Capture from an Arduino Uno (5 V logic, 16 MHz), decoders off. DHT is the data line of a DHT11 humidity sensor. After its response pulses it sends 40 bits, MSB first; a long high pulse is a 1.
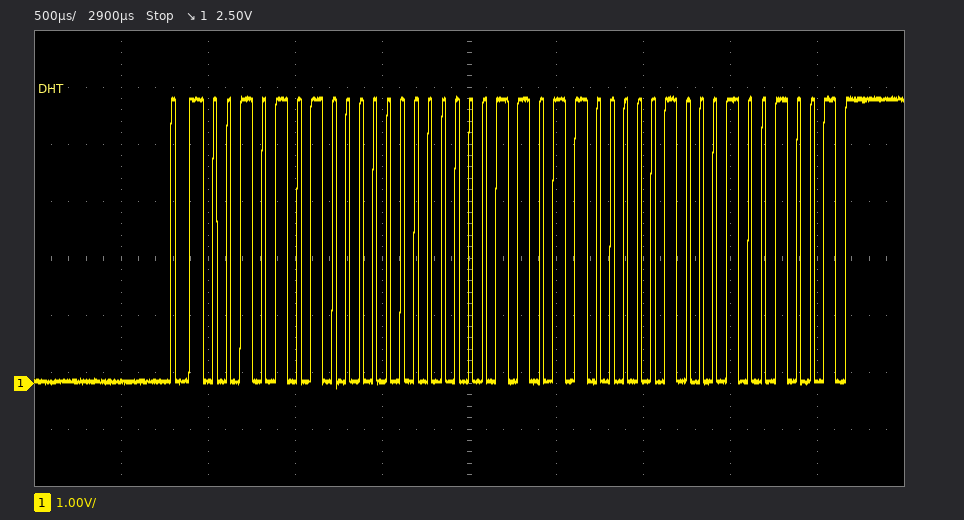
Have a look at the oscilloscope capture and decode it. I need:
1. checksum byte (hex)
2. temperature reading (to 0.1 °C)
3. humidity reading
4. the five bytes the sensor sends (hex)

0x49
27.4 °C
42 %
2A 00 1B 04 49
